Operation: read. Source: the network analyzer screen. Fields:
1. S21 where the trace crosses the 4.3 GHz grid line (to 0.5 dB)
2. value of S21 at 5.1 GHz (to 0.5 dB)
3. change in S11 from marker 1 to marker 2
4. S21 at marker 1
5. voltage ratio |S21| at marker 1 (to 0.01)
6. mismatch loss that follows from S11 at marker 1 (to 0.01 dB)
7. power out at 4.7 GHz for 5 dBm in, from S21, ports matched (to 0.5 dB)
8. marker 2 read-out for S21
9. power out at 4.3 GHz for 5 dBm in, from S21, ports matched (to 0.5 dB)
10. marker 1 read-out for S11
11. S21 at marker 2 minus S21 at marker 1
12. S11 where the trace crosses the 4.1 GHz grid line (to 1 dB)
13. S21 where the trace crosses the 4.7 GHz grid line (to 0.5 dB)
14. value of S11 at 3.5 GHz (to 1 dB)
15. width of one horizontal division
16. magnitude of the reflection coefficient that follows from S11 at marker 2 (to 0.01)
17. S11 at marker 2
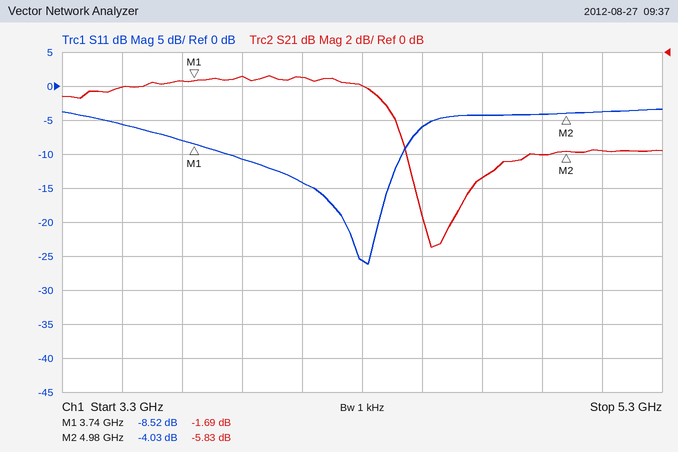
-2.0 dB
-6.0 dB
4.49 dB
-1.69 dB
0.82
0.66 dB
-2.5 dBm
-5.83 dB
3.0 dBm
-8.52 dB
-4.14 dB
-14 dB
-7.5 dB
-6 dB
200 MHz
0.63
-4.03 dB
